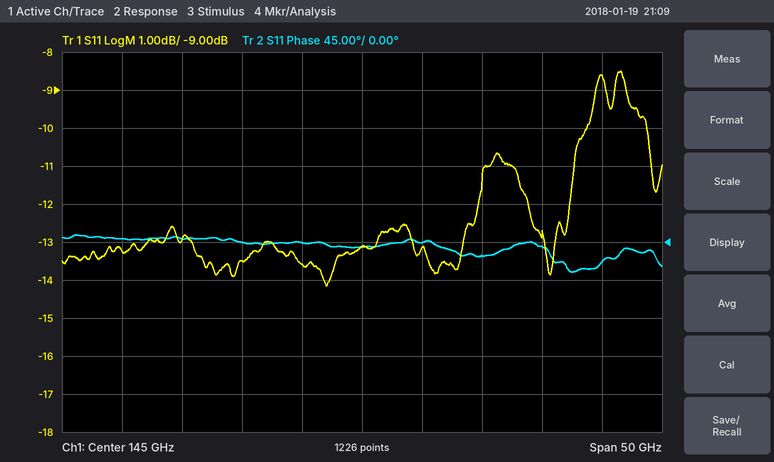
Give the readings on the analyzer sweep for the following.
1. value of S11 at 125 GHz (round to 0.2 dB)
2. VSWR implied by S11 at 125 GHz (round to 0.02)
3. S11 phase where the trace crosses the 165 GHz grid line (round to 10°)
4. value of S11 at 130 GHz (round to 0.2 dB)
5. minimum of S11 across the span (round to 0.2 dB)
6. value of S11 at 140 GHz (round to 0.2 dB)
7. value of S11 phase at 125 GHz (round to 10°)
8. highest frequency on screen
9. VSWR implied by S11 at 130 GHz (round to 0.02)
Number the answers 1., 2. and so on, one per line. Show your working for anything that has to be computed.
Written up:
1. -13.2 dB
2. |Γ| = 10^(-13.2/20) = 0.2188; VSWR = (1 + 0.2188)/(1 − 0.2188) ≈ 1.56
3. -20°
4. -13.0 dB
5. -14.2 dB
6. -13.6 dB
7. 0°
8. 170 GHz
9. |Γ| = 10^(-13/20) = 0.2239; VSWR = (1 + 0.2239)/(1 − 0.2239) ≈ 1.58
